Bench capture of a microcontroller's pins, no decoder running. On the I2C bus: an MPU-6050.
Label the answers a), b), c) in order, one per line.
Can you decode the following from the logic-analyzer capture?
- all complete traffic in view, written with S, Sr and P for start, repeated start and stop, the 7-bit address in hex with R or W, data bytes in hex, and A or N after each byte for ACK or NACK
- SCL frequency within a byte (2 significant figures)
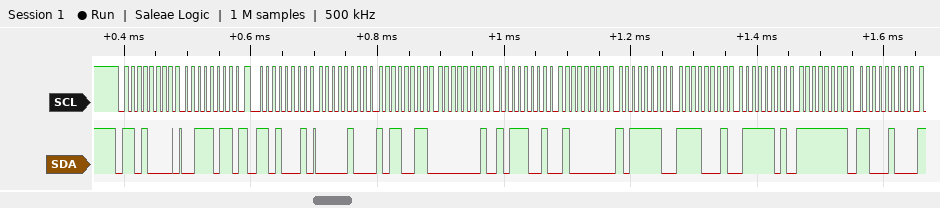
a) S 68W A 3B A Sr 68R A 04 A B3 A 01 A B9 A 40 A BE A F1 A 7D A FF A C4 A
b) 100 kHz
